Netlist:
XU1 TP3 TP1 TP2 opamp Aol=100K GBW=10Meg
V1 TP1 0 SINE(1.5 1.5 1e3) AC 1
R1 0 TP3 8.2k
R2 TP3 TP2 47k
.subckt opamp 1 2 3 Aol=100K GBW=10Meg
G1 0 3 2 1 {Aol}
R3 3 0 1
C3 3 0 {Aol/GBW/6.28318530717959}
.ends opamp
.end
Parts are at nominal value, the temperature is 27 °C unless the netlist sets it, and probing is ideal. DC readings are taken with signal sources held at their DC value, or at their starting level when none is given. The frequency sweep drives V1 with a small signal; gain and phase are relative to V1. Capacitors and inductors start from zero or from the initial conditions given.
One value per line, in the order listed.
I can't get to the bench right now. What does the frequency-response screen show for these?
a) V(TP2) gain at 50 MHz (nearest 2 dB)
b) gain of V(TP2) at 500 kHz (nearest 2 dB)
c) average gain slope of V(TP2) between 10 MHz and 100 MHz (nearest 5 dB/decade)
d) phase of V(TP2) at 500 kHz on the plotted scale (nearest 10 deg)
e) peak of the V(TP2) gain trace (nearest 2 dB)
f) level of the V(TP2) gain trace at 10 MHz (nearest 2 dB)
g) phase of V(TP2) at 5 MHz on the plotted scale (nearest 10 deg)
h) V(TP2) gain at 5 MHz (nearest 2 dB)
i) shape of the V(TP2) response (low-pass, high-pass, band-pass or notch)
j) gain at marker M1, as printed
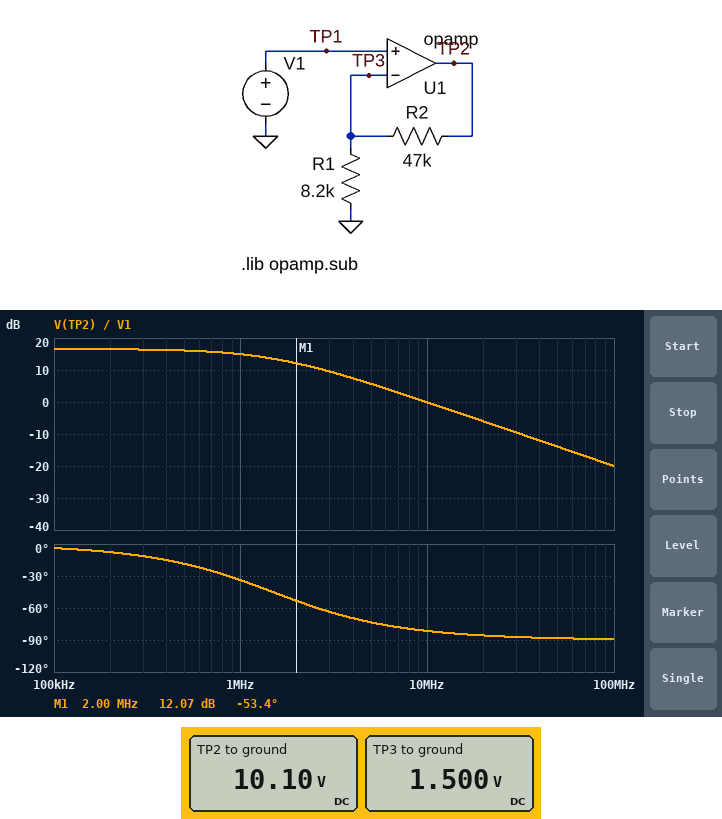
-14 dB
16 dB
-20 dB/decade
-20 deg
16 dB
0 dB
-70 deg
6 dB
low-pass
12.07 dB
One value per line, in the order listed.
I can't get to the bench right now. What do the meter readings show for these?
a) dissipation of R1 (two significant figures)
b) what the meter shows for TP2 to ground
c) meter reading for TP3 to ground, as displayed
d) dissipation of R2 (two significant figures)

270 µW
10.10 V
1.500 V
1.6 mW
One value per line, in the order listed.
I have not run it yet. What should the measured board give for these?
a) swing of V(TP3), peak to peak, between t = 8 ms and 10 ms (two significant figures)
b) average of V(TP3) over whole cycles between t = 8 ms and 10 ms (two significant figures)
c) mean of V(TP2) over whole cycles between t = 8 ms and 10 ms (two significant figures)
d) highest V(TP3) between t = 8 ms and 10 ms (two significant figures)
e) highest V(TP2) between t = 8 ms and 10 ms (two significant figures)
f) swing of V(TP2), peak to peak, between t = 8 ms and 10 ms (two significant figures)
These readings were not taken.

3.0 V
1.5 V
10 V
3.0 V
20 V
20 V
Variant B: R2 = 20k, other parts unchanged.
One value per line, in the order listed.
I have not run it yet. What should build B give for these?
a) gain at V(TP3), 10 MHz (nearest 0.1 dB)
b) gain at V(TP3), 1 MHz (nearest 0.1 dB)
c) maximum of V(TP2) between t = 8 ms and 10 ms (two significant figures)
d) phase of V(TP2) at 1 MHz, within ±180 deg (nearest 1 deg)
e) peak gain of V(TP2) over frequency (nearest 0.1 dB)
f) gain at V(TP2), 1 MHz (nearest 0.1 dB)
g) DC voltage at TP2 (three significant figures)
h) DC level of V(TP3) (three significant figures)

-11.1 dB
-0.5 dB
10 V
-19 deg
10.7 dB
10.2 dB
5.16 V
1.50 V
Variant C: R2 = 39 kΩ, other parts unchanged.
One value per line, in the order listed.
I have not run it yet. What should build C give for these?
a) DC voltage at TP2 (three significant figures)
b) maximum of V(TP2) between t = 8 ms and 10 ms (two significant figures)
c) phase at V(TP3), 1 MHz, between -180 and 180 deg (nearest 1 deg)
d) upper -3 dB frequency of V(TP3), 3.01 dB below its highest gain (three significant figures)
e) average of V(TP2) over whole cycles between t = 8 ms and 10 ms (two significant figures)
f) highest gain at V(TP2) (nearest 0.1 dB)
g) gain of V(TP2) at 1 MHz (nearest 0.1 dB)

8.63 V
17 V
-30 deg
1.74 MHz
8.6 V
15.2 dB
14.0 dB
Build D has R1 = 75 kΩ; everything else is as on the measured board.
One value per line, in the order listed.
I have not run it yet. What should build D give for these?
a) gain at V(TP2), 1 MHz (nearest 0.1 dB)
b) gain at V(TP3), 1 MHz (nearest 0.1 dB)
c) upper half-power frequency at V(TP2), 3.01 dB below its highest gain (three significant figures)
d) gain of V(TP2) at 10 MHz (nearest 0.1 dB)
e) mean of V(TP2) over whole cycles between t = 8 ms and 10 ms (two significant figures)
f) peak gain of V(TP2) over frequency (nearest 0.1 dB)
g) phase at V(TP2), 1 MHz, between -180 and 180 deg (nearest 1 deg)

4.1 dB
-0.1 dB
6.15 MHz
-1.4 dB
2.4 V
4.2 dB
-9 deg
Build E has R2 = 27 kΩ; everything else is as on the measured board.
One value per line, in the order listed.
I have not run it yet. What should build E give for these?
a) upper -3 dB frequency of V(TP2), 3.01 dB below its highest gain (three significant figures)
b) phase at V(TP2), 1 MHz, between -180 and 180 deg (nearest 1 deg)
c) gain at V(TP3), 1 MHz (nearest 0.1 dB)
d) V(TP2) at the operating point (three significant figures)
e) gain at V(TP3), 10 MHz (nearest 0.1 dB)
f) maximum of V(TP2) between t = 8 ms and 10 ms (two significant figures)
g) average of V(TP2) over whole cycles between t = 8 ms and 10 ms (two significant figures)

2.33 MHz
-23 deg
-0.7 dB
6.44 V
-12.9 dB
13 V
6.4 V
